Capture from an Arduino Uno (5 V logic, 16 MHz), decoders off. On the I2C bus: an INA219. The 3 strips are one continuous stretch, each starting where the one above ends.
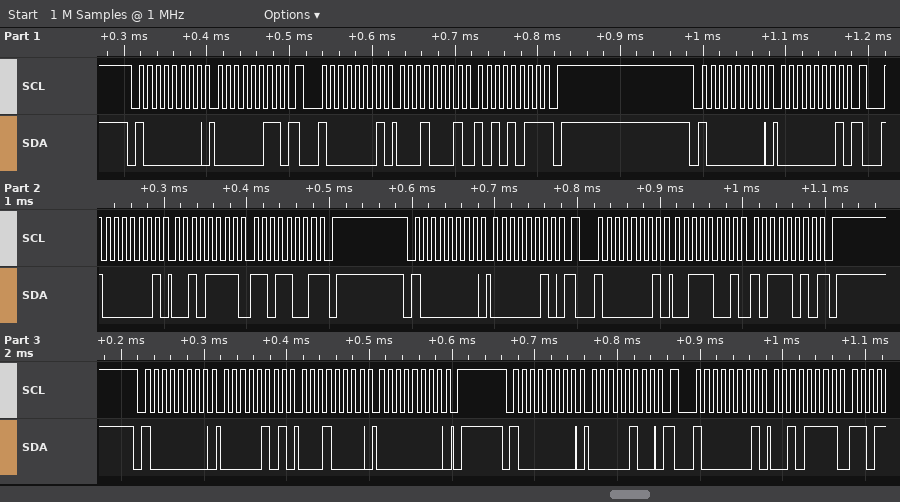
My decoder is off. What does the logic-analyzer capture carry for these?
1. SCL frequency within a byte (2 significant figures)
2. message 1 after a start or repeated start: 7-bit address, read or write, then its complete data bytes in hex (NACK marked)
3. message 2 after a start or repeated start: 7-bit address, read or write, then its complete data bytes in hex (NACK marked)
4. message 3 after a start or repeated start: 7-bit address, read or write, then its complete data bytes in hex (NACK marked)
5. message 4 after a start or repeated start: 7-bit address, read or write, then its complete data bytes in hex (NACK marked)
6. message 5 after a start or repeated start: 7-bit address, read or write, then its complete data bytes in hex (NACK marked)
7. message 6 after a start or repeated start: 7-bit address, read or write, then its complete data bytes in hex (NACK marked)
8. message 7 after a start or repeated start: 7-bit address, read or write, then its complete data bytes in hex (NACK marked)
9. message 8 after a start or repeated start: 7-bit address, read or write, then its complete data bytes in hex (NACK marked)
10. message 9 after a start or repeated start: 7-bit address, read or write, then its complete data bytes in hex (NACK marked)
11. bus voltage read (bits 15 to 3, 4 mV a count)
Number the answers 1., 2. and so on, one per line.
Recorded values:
1. 100 kHz
2. 0x40 write: 03
3. 0x40 read: 11 AB NACK
4. 0x40 write: 01
5. 0x40 read: 2F D9 NACK
6. 0x40 write: 02
7. 0x40 read: 39 BA NACK
8. 0x40 write: 05 10 00
9. 0x40 write: 04
10. 0x40 read: 2F
11. 7.388 V
